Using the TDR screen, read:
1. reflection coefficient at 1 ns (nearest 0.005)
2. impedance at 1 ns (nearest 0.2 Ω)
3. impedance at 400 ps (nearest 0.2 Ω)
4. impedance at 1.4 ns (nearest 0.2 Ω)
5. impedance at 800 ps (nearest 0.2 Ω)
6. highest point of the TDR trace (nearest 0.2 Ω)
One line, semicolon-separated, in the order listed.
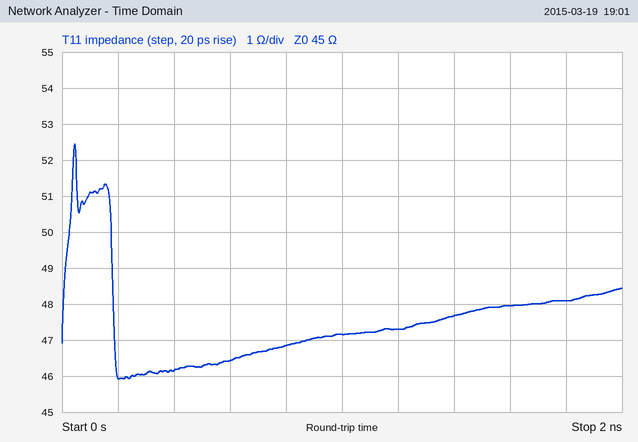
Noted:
+0.025; 47.2 Ω; 46.2 Ω; 47.6 Ω; 46.8 Ω; 52.4 Ω
